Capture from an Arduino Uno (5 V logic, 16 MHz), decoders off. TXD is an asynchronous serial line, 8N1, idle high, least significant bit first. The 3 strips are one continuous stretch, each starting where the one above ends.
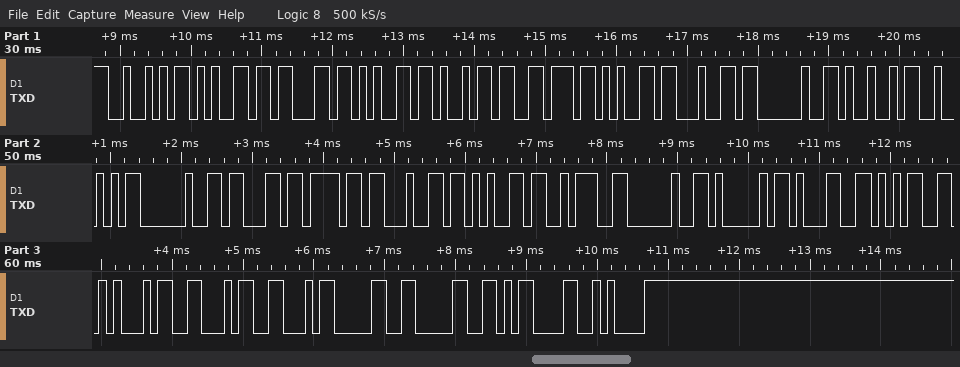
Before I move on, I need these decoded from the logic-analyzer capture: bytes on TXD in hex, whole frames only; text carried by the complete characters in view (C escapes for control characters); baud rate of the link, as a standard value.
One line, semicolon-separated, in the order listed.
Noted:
0x52 0x65 0x63 0x65 0x69 0x76 0x65 0x64 0x20 0x49 0x52 0x20 0x63 0x6F 0x64 0x65 0x3A 0x20 0x41 0x31 0x35 0x45 0x46 0x46 0x30 0x30 0x0D 0x0A; "Received IR code: A15EFF00\r\n"; 9600 baud
